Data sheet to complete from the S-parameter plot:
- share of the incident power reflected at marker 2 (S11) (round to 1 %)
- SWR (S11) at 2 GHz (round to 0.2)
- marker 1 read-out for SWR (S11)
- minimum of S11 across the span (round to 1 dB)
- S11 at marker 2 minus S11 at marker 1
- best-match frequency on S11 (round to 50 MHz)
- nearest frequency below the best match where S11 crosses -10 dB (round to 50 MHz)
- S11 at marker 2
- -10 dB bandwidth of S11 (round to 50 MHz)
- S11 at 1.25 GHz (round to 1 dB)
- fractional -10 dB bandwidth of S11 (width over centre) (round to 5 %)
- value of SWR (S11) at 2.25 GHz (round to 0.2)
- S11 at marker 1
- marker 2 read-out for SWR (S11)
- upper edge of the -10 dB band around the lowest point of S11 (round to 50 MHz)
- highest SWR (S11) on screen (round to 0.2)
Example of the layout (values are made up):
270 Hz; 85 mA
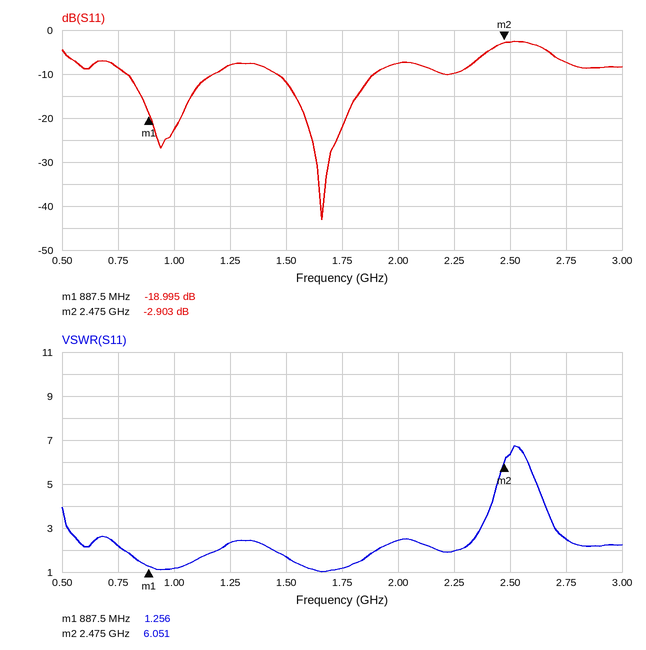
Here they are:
51 %; 2.4; 1.256; -43 dB; 16.092 dB; 1.65 GHz; 1.45 GHz; -2.903 dB; 450 MHz; -8 dB; 25 %; 2.0; -18.995 dB; 6.051; 1.90 GHz; 6.8
